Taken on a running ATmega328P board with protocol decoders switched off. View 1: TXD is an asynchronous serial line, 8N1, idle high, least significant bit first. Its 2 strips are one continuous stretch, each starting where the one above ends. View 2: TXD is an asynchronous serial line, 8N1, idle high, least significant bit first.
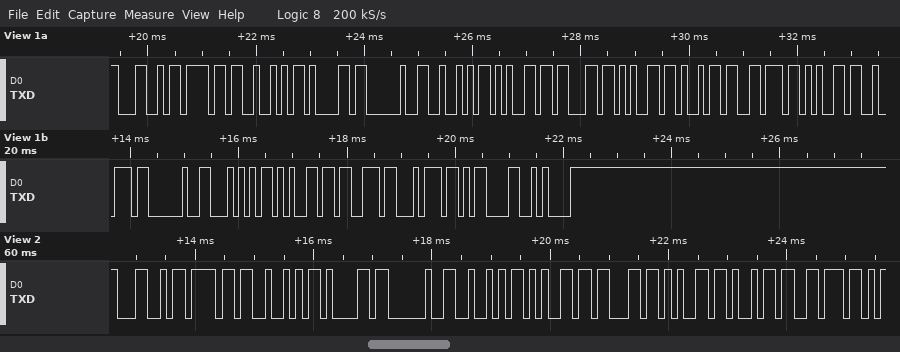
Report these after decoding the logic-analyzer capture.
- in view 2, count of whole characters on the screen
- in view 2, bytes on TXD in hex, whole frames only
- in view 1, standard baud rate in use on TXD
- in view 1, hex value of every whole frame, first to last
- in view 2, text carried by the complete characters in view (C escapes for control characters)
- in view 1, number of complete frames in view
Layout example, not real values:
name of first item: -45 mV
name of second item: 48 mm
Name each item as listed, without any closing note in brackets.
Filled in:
in view 2, count of whole characters on the screen: 11
in view 2, bytes on TXD in hex, whole frames only: 4C 6F 52 61 20 52 65 63 65 69 76
in view 1, standard baud rate in use on TXD: 9600 baud
in view 1, hex value of every whole frame, first to last: 4C 6F 52 61 20 52 65 63 65 69 76 65 72 20 54 65 73 74 0D 0A
in view 2, text carried by the complete characters in view: "LoRa Receiv"
in view 1, number of complete frames in view: 20
